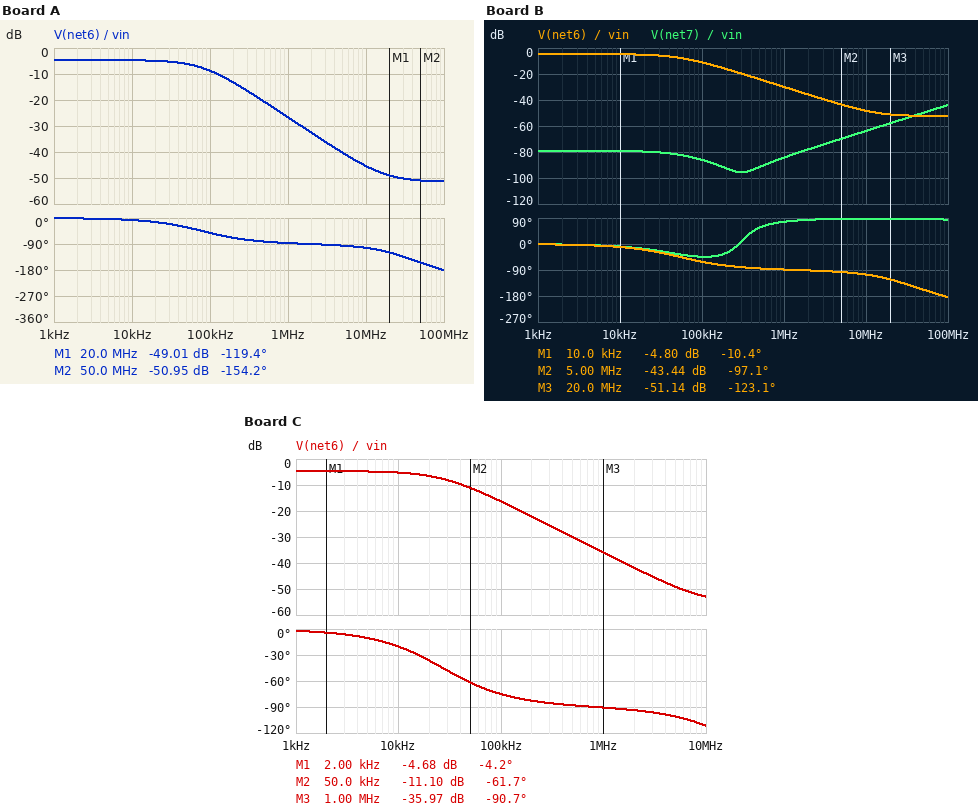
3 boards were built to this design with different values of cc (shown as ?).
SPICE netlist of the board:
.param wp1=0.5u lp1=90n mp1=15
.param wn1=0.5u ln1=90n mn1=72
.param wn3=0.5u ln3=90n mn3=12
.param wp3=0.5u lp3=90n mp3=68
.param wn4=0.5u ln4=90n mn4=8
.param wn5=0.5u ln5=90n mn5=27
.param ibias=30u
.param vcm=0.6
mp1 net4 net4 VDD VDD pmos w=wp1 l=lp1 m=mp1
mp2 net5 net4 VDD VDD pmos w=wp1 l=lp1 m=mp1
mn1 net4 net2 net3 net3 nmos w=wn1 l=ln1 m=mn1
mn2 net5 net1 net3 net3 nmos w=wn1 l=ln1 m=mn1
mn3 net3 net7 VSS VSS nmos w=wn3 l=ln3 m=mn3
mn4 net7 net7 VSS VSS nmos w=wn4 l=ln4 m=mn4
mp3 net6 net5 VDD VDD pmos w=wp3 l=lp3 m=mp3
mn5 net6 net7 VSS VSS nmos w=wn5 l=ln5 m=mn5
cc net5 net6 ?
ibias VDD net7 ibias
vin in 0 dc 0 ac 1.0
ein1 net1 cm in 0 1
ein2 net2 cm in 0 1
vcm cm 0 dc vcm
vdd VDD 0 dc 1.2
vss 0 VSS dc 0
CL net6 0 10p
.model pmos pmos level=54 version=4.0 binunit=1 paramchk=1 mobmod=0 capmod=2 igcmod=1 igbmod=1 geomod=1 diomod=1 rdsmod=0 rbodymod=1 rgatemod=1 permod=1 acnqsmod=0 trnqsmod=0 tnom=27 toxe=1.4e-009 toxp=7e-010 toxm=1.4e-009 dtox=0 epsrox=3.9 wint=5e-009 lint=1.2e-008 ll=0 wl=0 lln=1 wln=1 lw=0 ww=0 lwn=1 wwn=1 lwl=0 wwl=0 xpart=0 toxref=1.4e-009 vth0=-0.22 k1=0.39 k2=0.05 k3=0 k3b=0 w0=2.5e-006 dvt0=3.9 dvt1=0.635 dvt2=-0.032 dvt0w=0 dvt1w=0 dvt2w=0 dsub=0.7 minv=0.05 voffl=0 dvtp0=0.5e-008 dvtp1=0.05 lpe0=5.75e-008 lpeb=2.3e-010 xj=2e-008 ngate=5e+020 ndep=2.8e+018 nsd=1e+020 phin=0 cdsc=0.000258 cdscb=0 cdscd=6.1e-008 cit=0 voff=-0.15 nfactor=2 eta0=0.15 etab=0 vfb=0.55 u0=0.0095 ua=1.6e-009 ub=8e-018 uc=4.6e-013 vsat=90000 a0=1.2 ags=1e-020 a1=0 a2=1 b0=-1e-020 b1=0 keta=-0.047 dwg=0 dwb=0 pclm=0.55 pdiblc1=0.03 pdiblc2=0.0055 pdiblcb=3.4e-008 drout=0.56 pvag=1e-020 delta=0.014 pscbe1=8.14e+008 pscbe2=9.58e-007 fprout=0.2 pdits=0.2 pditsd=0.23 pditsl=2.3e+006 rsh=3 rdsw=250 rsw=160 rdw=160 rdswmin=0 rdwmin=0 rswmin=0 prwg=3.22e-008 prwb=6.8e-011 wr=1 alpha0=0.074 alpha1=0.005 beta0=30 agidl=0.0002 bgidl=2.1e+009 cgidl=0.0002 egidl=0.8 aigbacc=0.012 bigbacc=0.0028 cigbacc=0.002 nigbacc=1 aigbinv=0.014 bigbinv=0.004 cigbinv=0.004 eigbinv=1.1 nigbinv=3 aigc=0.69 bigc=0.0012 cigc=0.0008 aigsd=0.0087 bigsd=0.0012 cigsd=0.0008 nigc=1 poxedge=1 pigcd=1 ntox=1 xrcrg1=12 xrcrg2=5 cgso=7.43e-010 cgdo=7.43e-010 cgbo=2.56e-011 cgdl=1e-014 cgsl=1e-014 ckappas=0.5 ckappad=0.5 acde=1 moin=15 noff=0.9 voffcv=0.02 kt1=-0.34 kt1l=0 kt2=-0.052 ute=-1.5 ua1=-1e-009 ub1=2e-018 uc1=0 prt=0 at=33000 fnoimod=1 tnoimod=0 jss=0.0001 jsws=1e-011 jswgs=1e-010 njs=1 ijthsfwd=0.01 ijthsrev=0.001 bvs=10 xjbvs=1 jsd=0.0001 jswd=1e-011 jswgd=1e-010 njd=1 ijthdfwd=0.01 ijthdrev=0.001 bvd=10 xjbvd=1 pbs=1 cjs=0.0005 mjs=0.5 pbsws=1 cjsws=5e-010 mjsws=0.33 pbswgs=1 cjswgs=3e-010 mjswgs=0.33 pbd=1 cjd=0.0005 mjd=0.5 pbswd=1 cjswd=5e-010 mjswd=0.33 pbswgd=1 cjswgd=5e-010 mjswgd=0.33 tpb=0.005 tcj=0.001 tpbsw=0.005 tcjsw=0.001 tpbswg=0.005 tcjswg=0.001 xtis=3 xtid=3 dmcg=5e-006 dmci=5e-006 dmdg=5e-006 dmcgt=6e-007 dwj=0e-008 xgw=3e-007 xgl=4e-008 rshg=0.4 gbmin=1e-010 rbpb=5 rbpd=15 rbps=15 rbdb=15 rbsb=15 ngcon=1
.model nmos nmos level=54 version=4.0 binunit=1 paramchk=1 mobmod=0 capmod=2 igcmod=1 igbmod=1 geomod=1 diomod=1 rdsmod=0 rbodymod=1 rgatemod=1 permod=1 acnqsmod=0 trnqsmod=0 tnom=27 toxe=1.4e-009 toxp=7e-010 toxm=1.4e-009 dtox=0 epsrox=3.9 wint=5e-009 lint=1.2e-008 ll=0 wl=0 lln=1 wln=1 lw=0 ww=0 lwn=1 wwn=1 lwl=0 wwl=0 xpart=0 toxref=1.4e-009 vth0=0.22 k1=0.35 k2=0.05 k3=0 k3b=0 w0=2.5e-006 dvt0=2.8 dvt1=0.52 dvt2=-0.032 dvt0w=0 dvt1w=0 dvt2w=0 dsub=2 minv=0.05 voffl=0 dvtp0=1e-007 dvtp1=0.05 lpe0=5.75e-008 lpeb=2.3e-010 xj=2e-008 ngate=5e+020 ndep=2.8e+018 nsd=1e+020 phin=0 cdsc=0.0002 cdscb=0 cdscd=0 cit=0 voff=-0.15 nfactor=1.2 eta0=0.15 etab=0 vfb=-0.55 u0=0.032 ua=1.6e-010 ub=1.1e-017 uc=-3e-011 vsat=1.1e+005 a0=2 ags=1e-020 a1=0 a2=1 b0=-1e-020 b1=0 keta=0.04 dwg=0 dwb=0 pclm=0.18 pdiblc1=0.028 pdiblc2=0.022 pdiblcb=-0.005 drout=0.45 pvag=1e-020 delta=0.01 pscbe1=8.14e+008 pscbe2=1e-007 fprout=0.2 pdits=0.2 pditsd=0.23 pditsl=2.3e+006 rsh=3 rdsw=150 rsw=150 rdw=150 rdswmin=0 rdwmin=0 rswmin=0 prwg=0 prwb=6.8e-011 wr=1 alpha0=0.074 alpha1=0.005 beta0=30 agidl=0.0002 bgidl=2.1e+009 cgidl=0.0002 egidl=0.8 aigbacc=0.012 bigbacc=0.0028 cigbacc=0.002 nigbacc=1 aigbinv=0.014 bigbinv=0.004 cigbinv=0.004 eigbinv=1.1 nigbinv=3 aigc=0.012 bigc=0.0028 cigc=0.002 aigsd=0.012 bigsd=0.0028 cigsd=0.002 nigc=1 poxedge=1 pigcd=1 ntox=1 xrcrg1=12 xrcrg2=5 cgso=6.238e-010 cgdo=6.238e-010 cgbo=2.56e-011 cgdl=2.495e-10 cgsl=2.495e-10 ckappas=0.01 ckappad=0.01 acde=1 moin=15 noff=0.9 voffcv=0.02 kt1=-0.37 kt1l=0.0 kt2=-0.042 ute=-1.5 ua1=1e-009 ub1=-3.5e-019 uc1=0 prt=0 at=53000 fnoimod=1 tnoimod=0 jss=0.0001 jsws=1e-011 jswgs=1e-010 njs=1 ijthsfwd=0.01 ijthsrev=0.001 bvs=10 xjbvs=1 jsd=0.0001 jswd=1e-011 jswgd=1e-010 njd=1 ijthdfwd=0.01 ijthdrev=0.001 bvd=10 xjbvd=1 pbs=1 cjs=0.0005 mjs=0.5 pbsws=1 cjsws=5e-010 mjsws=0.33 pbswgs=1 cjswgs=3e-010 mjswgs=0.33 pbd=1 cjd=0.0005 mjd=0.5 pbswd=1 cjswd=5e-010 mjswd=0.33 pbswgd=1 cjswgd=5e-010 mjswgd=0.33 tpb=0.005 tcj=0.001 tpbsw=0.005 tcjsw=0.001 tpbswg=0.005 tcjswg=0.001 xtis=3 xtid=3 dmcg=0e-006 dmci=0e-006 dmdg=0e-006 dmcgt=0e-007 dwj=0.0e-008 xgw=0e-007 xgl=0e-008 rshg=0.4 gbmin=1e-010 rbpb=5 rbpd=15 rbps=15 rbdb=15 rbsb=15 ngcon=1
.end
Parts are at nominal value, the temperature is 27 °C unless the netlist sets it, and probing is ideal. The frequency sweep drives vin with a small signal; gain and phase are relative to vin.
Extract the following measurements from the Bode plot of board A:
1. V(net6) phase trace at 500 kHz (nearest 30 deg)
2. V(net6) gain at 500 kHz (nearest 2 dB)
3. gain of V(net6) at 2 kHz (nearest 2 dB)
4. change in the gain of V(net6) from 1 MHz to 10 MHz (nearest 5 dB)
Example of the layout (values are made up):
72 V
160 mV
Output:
-90 deg
-20 dB
-4 dB
-20 dB
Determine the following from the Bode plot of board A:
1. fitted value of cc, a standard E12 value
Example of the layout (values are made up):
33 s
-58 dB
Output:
2.2 pF
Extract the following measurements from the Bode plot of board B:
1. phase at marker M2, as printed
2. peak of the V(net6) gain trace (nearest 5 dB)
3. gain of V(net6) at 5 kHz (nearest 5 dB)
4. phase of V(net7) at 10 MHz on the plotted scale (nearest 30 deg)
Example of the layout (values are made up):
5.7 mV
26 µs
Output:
-97.1 deg
-5 dB
-5 dB
90 deg
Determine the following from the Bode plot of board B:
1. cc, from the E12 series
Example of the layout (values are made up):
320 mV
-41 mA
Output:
3.3 pF
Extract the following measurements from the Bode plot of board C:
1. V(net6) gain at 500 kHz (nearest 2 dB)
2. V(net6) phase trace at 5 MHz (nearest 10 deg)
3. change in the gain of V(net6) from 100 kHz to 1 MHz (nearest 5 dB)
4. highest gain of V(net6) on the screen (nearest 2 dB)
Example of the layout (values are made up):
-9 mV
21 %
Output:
-30 dB
-100 deg
-20 dB
-4 dB
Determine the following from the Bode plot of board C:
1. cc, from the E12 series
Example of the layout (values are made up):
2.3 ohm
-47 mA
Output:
6.8 pF
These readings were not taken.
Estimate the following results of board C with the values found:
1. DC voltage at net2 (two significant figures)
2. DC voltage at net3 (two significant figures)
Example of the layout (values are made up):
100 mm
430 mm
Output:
600 mV
340 mV
